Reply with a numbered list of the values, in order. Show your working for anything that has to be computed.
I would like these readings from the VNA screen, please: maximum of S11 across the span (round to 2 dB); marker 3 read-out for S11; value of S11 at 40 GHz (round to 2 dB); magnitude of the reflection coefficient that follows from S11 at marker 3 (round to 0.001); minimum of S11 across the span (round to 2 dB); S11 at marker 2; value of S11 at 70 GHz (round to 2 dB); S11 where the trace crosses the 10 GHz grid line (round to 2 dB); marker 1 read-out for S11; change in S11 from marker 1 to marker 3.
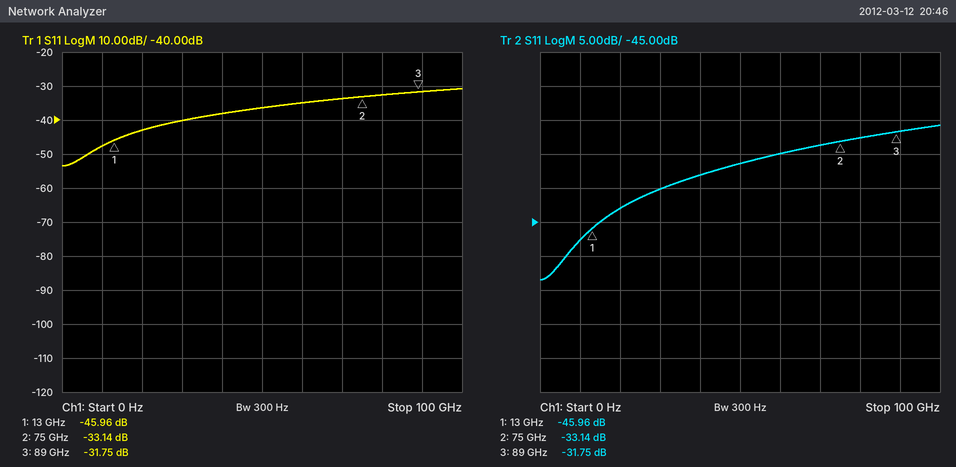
1. -30 dB
2. -31.75 dB
3. -38 dB
4. 10^(-31.75/20) ≈ 0.026
5. -54 dB
6. -33.14 dB
7. -34 dB
8. -48 dB
9. -45.96 dB
10. -31.75 − (-45.96) = 14.21 dB
